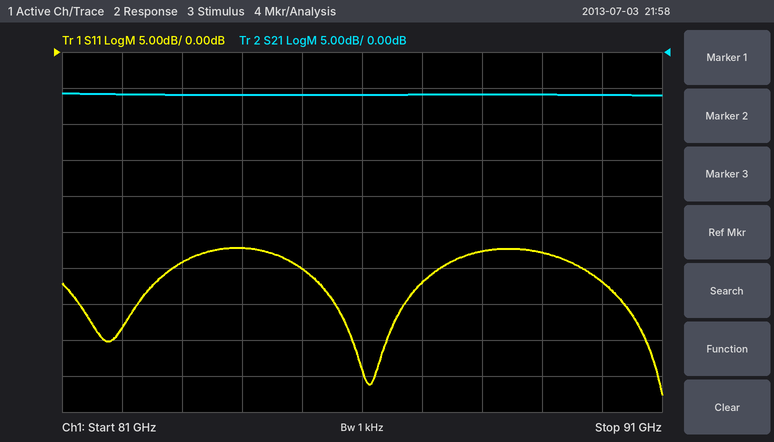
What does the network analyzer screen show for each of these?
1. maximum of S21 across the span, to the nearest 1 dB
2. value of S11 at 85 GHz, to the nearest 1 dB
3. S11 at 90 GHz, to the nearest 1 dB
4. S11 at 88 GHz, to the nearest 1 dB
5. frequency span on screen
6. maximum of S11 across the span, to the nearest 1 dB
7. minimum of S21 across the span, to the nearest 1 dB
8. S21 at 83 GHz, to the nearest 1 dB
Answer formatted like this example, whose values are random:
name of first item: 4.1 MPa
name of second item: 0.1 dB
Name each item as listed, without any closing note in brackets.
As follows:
maximum of S21 across the span, to the nearest 1 dB: -6 dB
value of S11 at 85 GHz, to the nearest 1 dB: -30 dB
S11 at 90 GHz, to the nearest 1 dB: -32 dB
S11 at 88 GHz, to the nearest 1 dB: -28 dB
frequency span on screen: 10 GHz
maximum of S11 across the span, to the nearest 1 dB: -27 dB
minimum of S21 across the span, to the nearest 1 dB: -6 dB
S21 at 83 GHz, to the nearest 1 dB: -6 dB
